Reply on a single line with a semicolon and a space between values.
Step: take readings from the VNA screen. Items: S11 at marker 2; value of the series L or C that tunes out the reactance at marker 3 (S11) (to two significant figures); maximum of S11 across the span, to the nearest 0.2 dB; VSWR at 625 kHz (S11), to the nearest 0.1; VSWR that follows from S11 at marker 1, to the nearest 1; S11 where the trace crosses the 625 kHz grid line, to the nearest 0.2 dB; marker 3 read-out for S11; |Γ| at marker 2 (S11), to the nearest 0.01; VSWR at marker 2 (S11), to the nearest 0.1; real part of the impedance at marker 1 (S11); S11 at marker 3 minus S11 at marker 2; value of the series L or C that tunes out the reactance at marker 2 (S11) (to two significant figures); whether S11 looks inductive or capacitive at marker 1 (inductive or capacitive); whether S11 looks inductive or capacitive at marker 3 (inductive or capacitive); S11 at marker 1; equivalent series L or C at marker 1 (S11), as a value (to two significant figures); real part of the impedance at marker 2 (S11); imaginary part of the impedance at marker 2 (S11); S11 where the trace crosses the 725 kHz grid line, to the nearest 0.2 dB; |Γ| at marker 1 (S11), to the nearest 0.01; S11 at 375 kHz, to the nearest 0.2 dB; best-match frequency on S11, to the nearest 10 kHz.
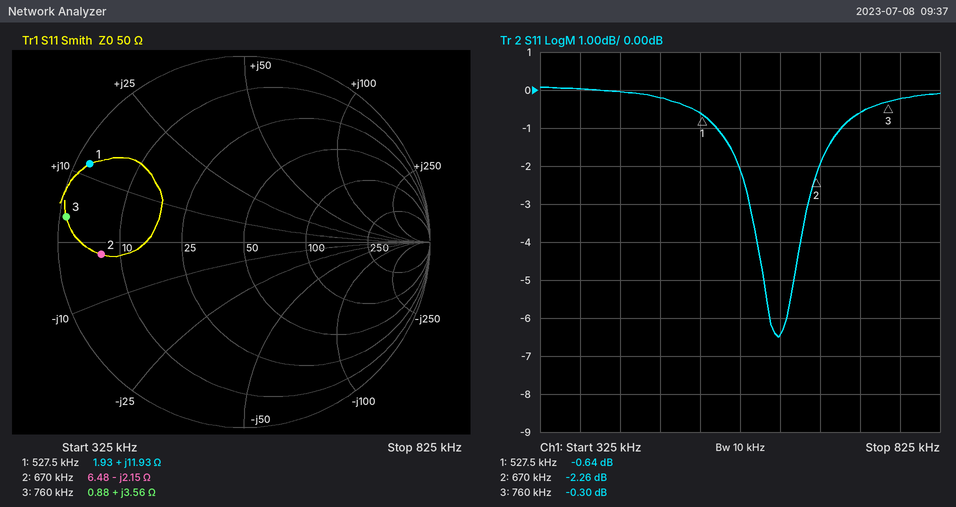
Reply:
-2.26 dB; 59 nF; 0.0 dB; 2.8; 27; -6.4 dB; -0.30 dB; 0.77; 7.7; 1.93 Ω; 1.96 dB; 510 nH; inductive; inductive; -0.64 dB; 3.6 µH; 6.48 Ω; -2.15 Ω; -0.6 dB; 0.93; 0.0 dB; 620 kHz
